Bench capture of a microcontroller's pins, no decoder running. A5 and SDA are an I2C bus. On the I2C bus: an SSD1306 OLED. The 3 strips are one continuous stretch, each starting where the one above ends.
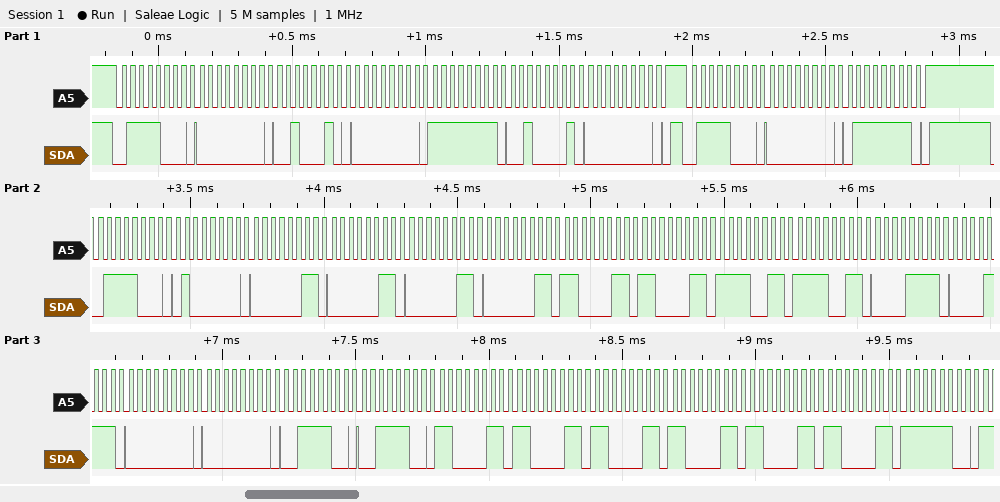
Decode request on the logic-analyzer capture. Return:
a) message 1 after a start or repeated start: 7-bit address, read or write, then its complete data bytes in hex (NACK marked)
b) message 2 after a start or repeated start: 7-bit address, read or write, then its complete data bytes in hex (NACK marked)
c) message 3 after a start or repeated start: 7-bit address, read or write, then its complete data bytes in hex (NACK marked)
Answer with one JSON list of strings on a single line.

["0x3C write: 00 22 00 FF 21 00", "0x3C write: 00 7F", "0x3C write: 40 03 03 03 03 C3 C3 F3 F3 0F 0F 00 00 3C 3C C3 C3 C3 C3 C3 C3 FC"]
